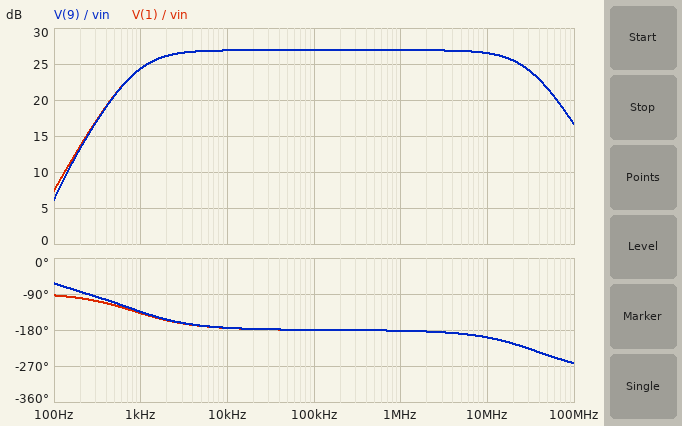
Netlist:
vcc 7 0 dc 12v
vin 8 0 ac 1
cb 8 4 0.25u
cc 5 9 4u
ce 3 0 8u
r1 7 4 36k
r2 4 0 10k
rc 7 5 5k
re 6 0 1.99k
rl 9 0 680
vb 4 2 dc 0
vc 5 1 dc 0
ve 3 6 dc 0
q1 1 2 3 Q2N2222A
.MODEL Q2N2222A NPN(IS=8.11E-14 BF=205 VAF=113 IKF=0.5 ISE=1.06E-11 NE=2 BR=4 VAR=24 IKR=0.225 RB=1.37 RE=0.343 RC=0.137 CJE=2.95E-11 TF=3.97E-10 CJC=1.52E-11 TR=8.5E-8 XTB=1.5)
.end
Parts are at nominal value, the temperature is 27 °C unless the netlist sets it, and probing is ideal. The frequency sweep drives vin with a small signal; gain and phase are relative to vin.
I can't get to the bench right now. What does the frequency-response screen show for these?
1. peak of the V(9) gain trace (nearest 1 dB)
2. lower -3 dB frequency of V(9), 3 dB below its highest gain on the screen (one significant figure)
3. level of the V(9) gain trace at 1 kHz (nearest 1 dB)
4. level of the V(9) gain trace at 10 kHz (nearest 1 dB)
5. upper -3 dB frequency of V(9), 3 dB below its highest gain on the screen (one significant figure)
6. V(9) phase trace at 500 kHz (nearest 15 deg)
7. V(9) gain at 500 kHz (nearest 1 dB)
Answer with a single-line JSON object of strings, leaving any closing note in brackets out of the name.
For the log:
{"peak of the V(9) gain trace": "27 dB", "lower -3 dB frequency of V(9), 3 dB below its highest gain on the screen": "900 Hz", "level of the V(9) gain trace at 1 kHz": "24 dB", "level of the V(9) gain trace at 10 kHz": "27 dB", "upper -3 dB frequency of V(9), 3 dB below its highest gain on the screen": "30 MHz", "V(9) phase trace at 500 kHz": "-180 deg", "V(9) gain at 500 kHz": "27 dB"}
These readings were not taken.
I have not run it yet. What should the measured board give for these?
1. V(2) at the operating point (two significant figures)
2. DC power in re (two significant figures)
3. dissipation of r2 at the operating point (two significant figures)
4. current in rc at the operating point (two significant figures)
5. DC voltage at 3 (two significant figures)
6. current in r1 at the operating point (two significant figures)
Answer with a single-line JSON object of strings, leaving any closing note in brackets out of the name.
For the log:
{"V(2) at the operating point": "2.6 V", "DC power in re": "1.9 mW", "dissipation of r2 at the operating point": "660 µW", "current in rc at the operating point": "980 µA", "DC voltage at 3": "2.0 V", "current in r1 at the operating point": "260 µA"}
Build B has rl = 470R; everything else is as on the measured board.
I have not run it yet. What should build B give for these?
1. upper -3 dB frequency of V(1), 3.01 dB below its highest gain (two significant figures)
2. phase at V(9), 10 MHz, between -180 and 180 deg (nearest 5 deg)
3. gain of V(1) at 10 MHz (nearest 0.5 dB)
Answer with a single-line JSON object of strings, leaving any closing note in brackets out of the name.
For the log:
{"upper -3 dB frequency of V(1), 3.01 dB below its highest gain": "44 MHz", "phase at V(9), 10 MHz, between -180 and 180 deg": "165 deg", "gain of V(1) at 10 MHz": "24.0 dB"}
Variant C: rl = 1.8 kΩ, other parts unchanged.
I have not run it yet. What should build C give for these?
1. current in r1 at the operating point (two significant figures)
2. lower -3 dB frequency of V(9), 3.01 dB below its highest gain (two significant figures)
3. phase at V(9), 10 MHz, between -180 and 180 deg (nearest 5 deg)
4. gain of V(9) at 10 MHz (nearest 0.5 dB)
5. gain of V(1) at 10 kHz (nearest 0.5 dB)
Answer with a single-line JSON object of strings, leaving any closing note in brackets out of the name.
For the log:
{"current in r1 at the operating point": "260 µA", "lower -3 dB frequency of V(9), 3.01 dB below its highest gain": "890 Hz", "phase at V(9), 10 MHz, between -180 and 180 deg": "145 deg", "gain of V(9) at 10 MHz": "32.0 dB", "gain of V(1) at 10 kHz": "33.5 dB"}
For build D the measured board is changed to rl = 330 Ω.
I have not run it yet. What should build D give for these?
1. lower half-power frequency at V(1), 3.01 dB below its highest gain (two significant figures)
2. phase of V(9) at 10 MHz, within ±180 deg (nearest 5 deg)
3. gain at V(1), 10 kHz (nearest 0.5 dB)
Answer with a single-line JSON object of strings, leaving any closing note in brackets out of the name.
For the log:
{"lower half-power frequency at V(1), 3.01 dB below its highest gain": "880 Hz", "phase of V(9) at 10 MHz, within ±180 deg": "170 deg", "gain at V(1), 10 kHz": "21.0 dB"}
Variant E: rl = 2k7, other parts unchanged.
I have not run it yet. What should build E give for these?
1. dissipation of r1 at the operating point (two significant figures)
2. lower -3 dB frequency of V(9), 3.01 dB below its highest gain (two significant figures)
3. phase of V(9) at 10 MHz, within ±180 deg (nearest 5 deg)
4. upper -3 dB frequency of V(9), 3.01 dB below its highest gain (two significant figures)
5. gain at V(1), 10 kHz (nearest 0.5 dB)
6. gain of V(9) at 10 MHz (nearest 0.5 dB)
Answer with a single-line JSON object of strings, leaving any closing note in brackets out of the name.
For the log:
{"dissipation of r1 at the operating point": "2.5 mW", "lower -3 dB frequency of V(9), 3.01 dB below its highest gain": "890 Hz", "phase of V(9) at 10 MHz, within ±180 deg": "135 deg", "upper -3 dB frequency of V(9), 3.01 dB below its highest gain": "11 MHz", "gain at V(1), 10 kHz": "36.0 dB", "gain of V(9) at 10 MHz": "33.5 dB"}
